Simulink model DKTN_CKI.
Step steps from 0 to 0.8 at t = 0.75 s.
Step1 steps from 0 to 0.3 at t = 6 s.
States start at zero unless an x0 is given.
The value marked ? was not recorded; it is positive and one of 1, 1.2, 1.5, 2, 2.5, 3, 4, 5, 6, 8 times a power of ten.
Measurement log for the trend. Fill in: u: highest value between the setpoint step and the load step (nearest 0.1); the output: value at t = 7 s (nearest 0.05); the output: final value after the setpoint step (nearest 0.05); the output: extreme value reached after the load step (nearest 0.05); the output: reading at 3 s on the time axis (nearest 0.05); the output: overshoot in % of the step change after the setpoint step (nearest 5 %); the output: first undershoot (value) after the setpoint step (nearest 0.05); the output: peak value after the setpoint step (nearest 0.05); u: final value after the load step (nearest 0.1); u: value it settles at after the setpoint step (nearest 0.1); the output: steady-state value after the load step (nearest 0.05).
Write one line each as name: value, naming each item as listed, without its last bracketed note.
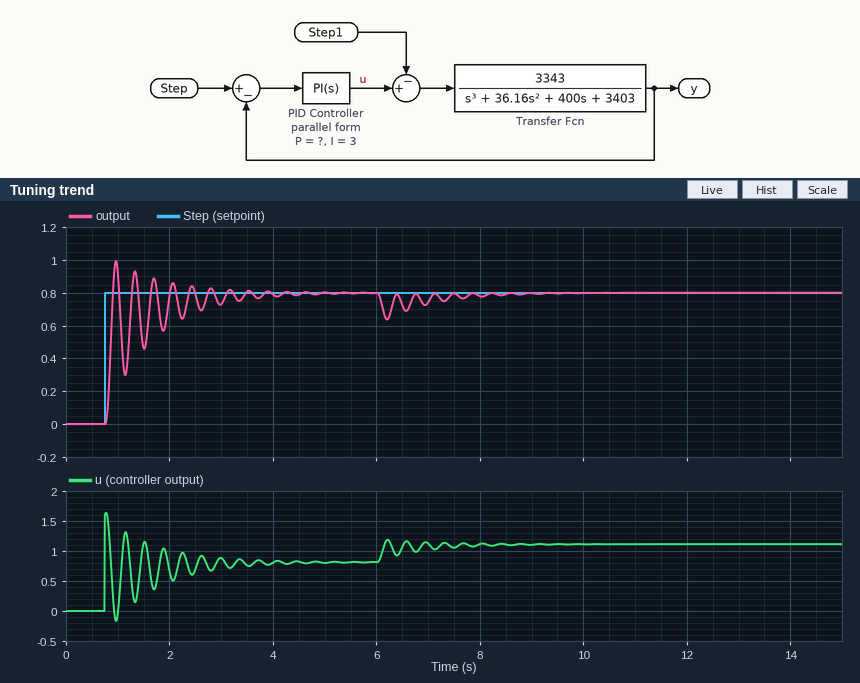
u: highest value between the setpoint step and the load step: 1.6
the output: value at t = 7 s: 0.75
the output: final value after the setpoint step: 0.80
the output: extreme value reached after the load step: 0.65
the output: reading at 3 s on the time axis: 0.75
the output: overshoot in % of the step change after the setpoint step: 25 %
the output: first undershoot (value) after the setpoint step: 0.30
the output: peak value after the setpoint step: 1.00
u: final value after the load step: 1.1
u: value it settles at after the setpoint step: 0.8
the output: steady-state value after the load step: 0.80
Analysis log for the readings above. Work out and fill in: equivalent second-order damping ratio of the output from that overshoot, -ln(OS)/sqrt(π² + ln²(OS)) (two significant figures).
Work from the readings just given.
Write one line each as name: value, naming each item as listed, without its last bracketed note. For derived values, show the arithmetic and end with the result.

equivalent second-order damping ratio of the output from that overshoot, -ln(OS)/sqrt(π² + ln²(OS)): ln(0.25) = -1.386; 1.386 / sqrt(9.870 + 1.922) = 0.40
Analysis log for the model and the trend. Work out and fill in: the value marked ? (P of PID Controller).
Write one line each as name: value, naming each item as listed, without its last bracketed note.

the value marked ?: 2
